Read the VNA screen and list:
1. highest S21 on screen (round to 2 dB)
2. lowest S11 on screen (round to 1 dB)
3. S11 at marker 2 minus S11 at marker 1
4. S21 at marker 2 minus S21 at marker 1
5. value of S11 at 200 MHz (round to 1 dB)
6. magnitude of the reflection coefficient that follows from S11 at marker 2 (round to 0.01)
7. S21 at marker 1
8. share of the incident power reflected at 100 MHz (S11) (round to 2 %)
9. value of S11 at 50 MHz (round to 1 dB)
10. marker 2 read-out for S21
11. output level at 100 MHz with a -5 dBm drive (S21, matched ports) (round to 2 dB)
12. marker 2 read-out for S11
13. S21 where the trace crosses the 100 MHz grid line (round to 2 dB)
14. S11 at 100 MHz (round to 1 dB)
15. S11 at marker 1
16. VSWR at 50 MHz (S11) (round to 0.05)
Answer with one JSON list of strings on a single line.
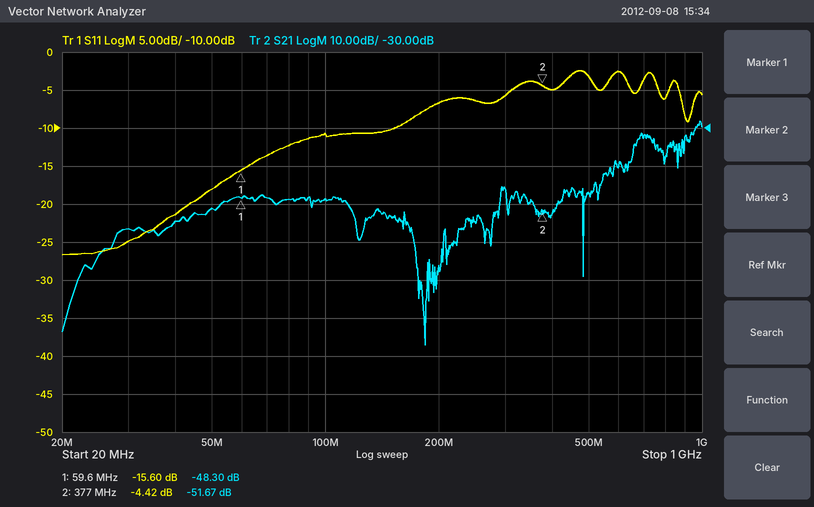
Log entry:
["-28 dB", "-27 dB", "11.18 dB", "-3.37 dB", "-7 dB", "0.60", "-48.30 dB", "8 %", "-18 dB", "-51.67 dB", "-54 dBm", "-4.42 dB", "-48 dB", "-11 dB", "-15.60 dB", "1.30"]
